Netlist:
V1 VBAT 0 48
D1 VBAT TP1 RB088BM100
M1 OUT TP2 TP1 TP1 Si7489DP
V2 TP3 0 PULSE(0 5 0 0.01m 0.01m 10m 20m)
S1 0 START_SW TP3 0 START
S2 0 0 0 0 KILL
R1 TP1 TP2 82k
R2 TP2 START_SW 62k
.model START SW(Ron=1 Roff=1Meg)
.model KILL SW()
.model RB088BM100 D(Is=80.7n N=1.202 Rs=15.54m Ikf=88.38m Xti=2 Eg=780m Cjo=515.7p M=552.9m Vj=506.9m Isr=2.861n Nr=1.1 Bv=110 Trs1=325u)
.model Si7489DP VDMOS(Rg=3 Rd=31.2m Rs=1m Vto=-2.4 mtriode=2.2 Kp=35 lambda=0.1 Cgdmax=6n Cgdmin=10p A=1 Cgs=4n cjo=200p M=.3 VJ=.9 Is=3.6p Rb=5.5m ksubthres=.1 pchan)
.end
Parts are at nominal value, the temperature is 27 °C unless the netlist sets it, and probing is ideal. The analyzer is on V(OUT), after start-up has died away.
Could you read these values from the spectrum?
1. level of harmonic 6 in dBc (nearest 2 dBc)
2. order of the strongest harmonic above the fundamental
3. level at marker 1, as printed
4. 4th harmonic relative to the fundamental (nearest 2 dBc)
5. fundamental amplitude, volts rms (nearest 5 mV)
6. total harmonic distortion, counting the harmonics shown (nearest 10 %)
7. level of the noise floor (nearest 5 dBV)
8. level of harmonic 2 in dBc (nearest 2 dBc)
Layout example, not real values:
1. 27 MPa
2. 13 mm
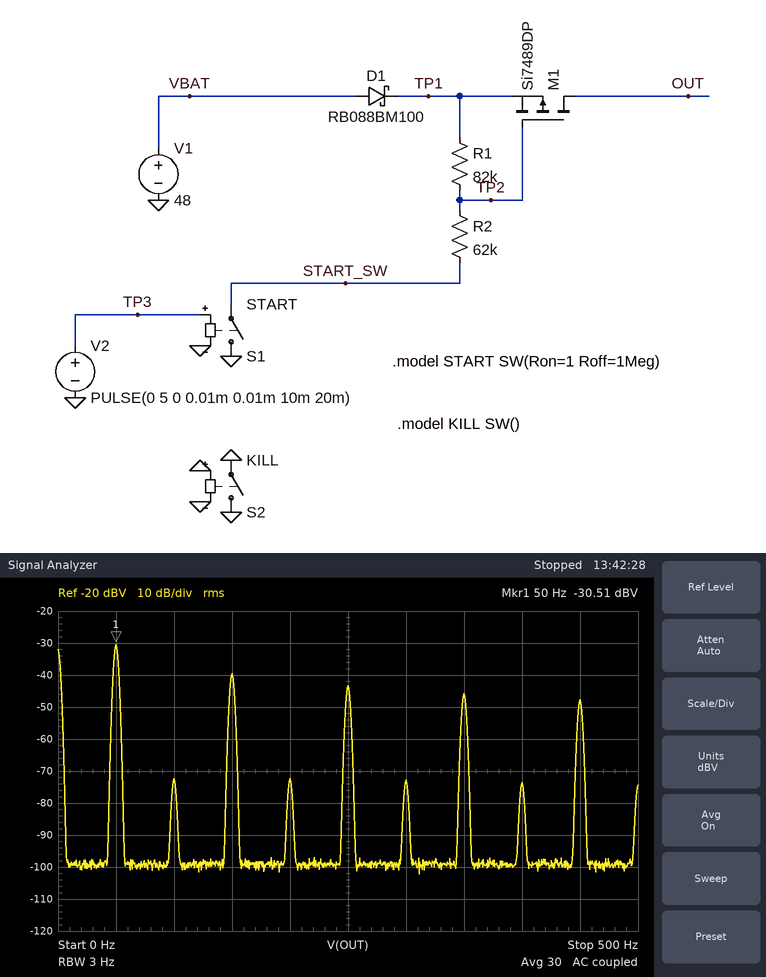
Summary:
1. -42 dBc
2. 3
3. -30.51 dBV
4. -42 dBc
5. 30 mV
6. 50 %
7. -100 dBV
8. -42 dBc
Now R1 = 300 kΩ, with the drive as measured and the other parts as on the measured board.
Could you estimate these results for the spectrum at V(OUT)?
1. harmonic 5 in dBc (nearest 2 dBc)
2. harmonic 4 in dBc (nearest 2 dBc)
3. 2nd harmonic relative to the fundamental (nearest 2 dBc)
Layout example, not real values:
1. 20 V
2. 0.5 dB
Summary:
1. -10 dBc
2. -28 dBc
3. -24 dBc
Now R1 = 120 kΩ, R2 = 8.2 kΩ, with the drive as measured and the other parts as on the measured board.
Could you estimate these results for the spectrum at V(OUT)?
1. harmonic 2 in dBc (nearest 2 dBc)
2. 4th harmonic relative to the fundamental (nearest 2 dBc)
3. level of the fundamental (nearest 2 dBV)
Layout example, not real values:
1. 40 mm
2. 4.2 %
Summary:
1. -24 dBc
2. -26 dBc
3. -30 dBV
